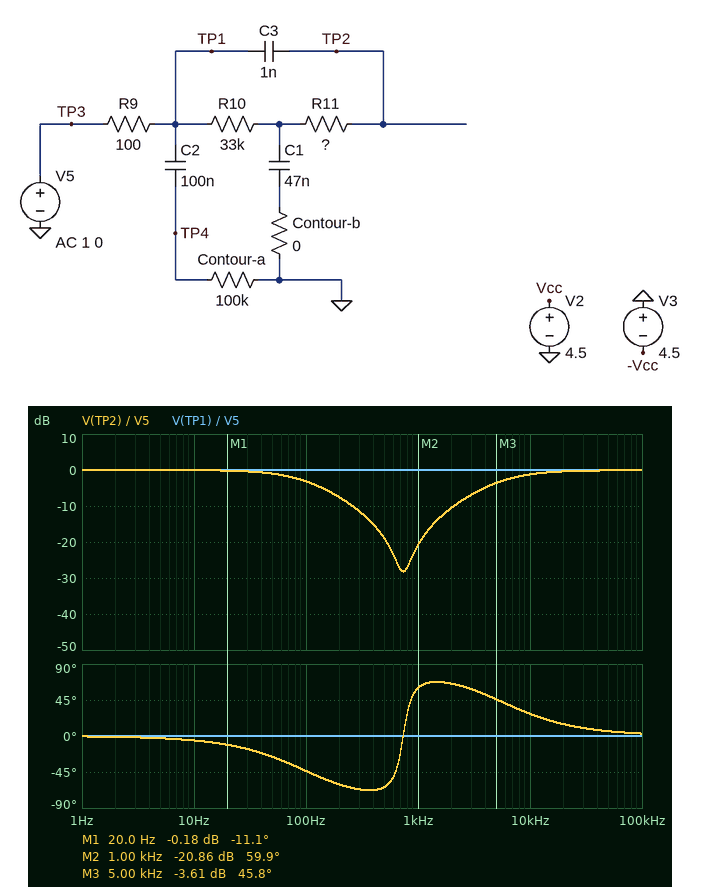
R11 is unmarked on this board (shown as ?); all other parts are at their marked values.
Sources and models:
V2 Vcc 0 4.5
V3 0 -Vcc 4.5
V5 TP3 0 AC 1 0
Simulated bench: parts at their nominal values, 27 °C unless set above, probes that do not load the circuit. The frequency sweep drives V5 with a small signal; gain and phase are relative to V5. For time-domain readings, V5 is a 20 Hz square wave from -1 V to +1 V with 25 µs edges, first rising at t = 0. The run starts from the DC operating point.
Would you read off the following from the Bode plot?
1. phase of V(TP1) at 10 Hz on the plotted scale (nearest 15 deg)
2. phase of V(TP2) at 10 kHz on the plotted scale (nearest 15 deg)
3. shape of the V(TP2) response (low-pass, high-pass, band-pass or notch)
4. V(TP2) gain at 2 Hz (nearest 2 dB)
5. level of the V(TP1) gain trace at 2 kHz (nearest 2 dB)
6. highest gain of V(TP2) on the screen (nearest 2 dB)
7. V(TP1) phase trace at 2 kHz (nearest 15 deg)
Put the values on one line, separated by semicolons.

0 deg; 30 deg; notch; 0 dB; 0 dB; 0 dB; 0 deg
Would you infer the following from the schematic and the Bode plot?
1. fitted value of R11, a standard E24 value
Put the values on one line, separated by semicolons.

30 kΩ
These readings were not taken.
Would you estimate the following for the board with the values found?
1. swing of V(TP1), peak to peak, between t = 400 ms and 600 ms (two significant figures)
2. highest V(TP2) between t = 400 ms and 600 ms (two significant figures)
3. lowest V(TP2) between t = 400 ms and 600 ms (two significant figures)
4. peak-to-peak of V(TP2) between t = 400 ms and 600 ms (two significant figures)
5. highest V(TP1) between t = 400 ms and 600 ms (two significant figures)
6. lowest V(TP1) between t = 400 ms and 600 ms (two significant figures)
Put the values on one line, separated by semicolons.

2.0 V; 1.0 V; -1.0 V; 2.0 V; 1.0 V; -1.0 V
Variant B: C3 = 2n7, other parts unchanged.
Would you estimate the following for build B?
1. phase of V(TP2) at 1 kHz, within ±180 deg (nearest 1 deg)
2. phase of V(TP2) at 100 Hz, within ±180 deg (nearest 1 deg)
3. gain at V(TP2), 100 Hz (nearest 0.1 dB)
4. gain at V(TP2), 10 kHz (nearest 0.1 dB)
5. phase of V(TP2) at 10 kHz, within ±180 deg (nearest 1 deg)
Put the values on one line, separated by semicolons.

55 deg; -42 deg; -3.6 dB; -0.3 dB; 11 deg
